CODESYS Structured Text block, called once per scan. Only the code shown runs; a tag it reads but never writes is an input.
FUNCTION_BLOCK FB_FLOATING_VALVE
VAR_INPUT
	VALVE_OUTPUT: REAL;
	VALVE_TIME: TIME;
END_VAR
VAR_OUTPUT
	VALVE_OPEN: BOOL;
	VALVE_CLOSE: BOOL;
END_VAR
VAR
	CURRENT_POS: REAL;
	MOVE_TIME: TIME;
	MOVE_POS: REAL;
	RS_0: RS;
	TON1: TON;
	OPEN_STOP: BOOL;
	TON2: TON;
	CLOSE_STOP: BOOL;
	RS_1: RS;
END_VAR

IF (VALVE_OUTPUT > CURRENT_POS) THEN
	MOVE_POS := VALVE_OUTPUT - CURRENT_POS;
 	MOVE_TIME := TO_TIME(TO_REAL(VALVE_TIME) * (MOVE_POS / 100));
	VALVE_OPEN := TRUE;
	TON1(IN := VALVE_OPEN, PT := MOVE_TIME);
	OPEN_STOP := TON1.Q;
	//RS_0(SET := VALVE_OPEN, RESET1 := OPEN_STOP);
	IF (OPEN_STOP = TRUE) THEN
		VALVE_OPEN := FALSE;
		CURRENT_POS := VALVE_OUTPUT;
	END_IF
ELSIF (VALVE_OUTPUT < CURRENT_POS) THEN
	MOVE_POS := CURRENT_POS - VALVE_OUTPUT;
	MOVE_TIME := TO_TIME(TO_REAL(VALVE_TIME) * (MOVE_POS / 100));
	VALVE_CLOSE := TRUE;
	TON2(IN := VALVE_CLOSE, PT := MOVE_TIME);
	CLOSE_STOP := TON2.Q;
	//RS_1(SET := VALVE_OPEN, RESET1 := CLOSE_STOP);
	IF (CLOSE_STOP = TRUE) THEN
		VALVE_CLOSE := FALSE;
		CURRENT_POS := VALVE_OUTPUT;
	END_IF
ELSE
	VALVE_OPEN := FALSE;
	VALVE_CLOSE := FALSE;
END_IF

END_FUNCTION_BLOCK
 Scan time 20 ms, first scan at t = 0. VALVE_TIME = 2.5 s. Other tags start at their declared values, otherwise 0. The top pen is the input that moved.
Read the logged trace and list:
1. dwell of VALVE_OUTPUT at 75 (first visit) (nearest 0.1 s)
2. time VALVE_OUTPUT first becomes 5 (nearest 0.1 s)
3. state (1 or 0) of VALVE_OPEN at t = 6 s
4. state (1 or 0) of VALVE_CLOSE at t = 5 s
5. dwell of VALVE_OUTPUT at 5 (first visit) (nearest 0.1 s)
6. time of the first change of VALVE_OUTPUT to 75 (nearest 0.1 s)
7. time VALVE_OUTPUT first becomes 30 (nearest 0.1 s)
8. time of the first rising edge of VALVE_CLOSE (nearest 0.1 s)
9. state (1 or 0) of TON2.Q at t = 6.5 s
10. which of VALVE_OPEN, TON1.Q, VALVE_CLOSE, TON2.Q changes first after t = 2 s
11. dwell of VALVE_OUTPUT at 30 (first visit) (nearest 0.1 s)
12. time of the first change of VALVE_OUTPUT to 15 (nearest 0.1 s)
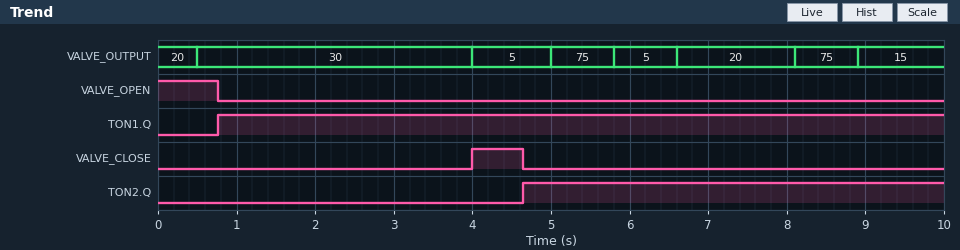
0.8 s
4.0 s
0
0
1.0 s
5.0 s
0.5 s
4.0 s
1
VALVE_CLOSE
3.5 s
8.9 s
